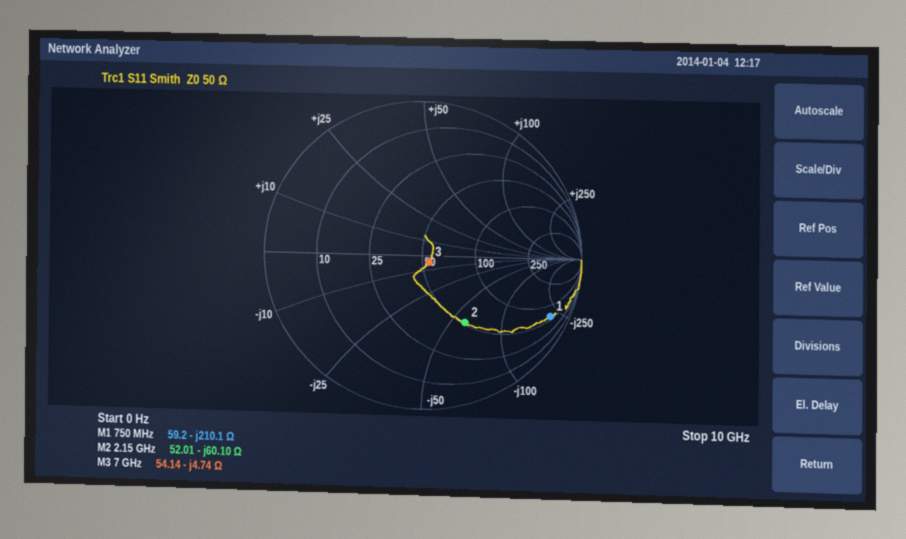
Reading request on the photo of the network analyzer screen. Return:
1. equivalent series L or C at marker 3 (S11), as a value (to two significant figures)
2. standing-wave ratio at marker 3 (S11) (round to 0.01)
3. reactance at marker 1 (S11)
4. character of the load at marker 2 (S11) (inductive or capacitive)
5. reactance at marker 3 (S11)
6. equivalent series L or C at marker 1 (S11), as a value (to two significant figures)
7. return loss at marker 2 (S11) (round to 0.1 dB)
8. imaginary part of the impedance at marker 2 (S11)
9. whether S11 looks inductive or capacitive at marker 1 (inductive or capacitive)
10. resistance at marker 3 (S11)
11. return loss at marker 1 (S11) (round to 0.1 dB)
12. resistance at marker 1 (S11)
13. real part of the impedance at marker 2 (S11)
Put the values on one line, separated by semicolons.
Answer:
4.8 pF; 1.13; -210.1 Ω; capacitive; -4.74 Ω; 1.0 pF; 5.9 dB; -60.10 Ω; capacitive; 54.14 Ω; 1.0 dB; 59.2 Ω; 52.01 Ω
